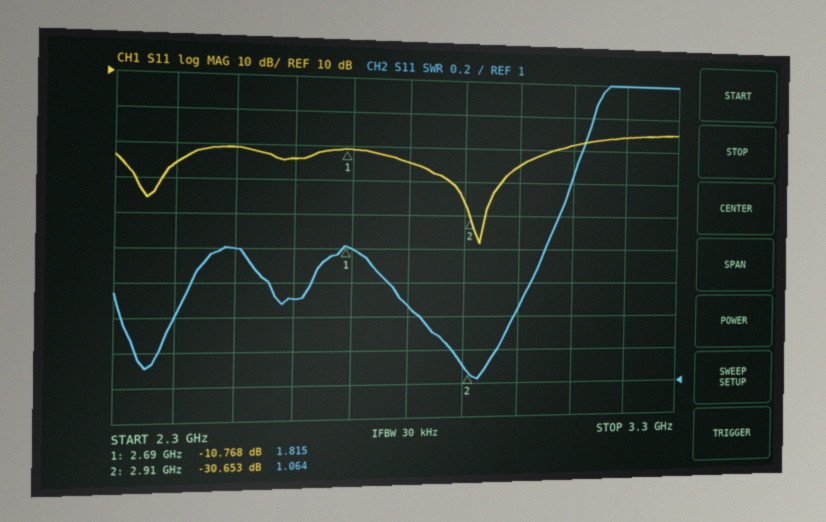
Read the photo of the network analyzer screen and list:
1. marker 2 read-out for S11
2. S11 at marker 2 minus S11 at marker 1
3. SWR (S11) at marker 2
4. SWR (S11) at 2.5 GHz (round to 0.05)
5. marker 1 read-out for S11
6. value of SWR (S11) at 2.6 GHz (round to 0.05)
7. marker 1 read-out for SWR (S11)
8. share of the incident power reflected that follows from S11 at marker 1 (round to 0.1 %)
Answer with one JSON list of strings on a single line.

["-30.653 dB", "-19.885 dB", "1.064", "1.80", "-10.768 dB", "1.50", "1.815", "8.4 %"]
